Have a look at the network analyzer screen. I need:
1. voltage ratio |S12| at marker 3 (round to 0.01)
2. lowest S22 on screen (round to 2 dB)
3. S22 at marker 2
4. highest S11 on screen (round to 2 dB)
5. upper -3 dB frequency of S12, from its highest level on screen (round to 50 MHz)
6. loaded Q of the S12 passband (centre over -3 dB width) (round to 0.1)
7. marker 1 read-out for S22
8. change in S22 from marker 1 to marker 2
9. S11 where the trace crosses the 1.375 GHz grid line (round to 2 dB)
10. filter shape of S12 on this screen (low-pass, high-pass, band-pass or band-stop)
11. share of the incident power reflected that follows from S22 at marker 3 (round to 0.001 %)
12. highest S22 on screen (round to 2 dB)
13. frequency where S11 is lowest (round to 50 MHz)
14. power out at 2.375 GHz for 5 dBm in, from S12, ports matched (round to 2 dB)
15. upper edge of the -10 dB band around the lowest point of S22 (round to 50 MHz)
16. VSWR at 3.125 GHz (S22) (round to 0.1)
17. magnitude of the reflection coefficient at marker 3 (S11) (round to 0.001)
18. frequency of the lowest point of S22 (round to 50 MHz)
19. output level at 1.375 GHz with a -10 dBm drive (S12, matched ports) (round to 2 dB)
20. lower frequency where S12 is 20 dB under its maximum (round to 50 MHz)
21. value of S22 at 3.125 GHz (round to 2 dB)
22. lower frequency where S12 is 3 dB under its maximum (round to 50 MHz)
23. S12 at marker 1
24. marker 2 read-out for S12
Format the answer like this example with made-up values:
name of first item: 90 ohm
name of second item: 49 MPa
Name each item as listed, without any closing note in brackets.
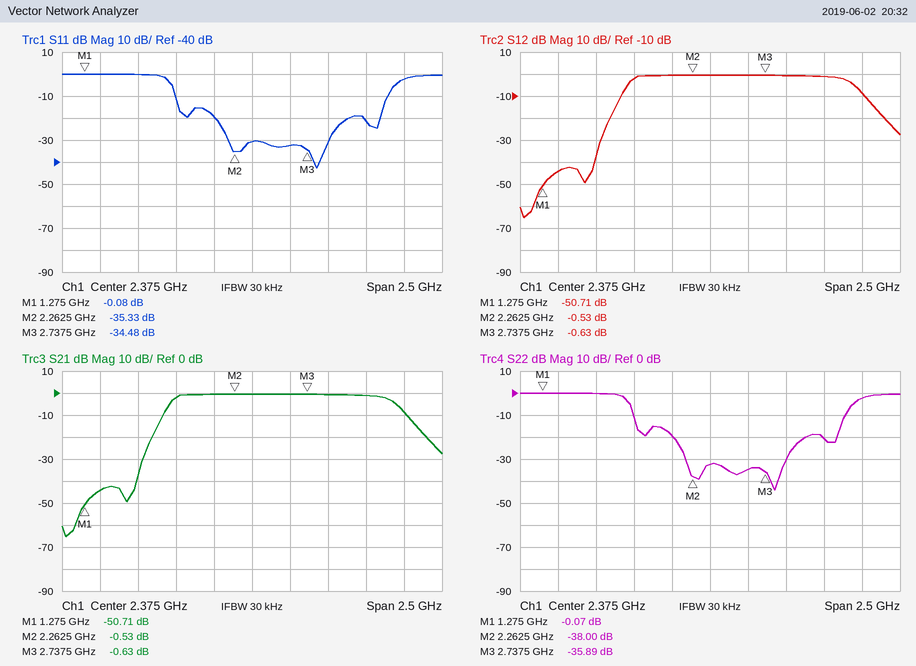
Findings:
voltage ratio |S12| at marker 3: 0.93
lowest S22 on screen: -44 dB
S22 at marker 2: -38.00 dB
highest S11 on screen: 0 dB
upper -3 dB frequency of S12, from its highest level on screen: 3.30 GHz
loaded Q of the S12 passband (centre over -3 dB width): 1.8
marker 1 read-out for S22: -0.07 dB
change in S22 from marker 1 to marker 2: -37.93 dB
S11 where the trace crosses the 1.375 GHz grid line: 0 dB
filter shape of S12 on this screen: band-pass
share of the incident power reflected that follows from S22 at marker 3: 0.026 %
highest S22 on screen: 0 dB
frequency where S11 is lowest: 2.80 GHz
power out at 2.375 GHz for 5 dBm in, from S12, ports matched: 4 dBm
upper edge of the -10 dB band around the lowest point of S22: 3.25 GHz
VSWR at 3.125 GHz (S22): 1.2
magnitude of the reflection coefficient at marker 3 (S11): 0.019
frequency of the lowest point of S22: 2.80 GHz
output level at 1.375 GHz with a -10 dBm drive (S12, matched ports): -54 dBm
lower frequency where S12 is 20 dB under its maximum: 1.70 GHz
value of S22 at 3.125 GHz: -20 dB
lower frequency where S12 is 3 dB under its maximum: 1.85 GHz
S12 at marker 1: -50.71 dB
marker 2 read-out for S12: -0.53 dB
